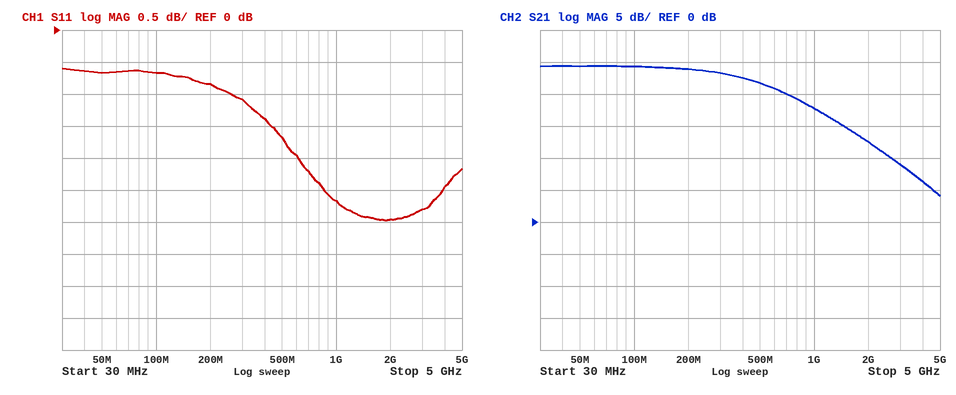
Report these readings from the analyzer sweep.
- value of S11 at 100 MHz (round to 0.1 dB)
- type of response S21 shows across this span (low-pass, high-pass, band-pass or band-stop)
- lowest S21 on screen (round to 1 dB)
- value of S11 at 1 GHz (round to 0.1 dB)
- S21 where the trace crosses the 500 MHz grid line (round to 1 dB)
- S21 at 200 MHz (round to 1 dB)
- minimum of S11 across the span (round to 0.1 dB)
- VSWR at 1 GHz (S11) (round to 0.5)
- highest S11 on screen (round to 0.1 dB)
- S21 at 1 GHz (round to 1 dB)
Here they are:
-0.7 dB
low-pass
4 dB
-2.7 dB
22 dB
24 dB
-3.0 dB
6.5
-0.6 dB
18 dB
